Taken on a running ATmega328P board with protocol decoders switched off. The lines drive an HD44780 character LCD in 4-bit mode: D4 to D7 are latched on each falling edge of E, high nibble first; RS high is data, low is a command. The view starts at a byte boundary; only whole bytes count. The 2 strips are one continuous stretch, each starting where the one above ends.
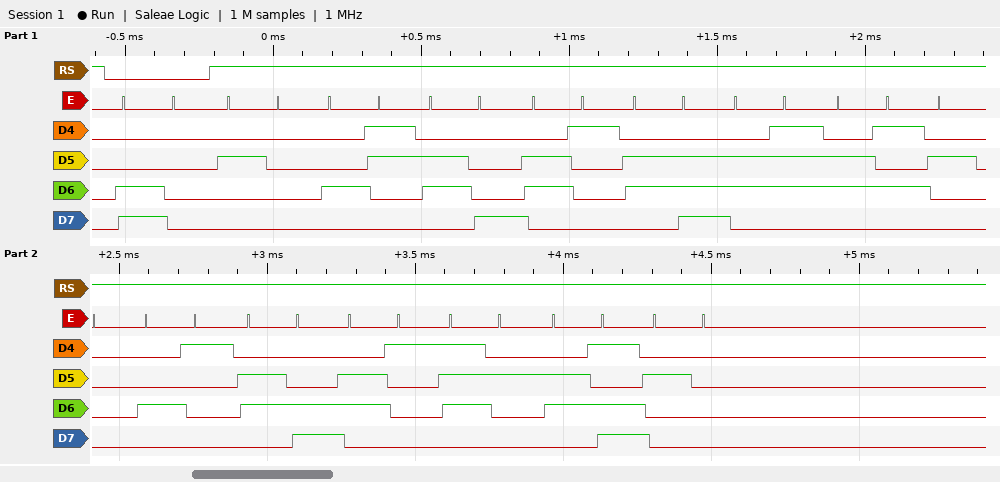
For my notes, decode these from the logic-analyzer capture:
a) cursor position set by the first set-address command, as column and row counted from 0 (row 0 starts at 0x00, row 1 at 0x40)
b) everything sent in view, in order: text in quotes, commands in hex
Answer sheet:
column 0, row 1
0xC0 " Change Alarm "
